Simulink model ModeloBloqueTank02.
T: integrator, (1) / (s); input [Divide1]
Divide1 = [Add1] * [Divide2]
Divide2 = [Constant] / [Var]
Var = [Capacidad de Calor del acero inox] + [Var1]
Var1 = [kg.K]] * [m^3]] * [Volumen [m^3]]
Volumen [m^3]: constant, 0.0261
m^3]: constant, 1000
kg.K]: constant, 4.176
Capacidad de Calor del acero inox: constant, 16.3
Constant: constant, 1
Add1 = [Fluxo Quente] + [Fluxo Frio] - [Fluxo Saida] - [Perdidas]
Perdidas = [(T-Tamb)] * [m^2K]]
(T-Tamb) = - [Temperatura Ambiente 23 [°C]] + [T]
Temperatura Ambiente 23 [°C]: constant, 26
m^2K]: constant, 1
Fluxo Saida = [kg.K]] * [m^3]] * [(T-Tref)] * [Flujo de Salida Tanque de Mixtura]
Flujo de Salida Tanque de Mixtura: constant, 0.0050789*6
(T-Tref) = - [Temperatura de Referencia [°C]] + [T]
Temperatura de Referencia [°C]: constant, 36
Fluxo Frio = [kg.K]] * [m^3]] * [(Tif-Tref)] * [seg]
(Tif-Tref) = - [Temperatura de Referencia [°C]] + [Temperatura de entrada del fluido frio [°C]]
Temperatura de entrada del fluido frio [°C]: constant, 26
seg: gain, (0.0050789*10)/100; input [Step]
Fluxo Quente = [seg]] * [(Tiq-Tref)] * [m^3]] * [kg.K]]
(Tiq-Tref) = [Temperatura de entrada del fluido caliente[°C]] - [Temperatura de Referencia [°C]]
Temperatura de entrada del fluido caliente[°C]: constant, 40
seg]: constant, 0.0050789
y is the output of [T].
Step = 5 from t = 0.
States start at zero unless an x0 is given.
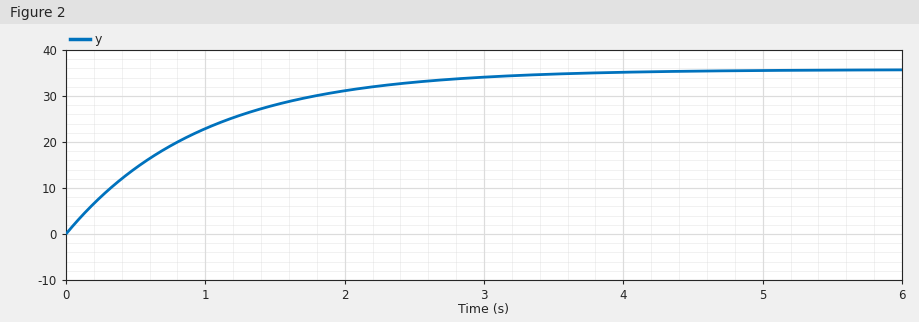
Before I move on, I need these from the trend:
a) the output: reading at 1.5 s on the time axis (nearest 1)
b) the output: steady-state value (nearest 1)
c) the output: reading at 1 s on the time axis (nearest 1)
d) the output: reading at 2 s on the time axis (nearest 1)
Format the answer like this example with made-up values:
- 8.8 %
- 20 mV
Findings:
- 28
- 36
- 23
- 31
